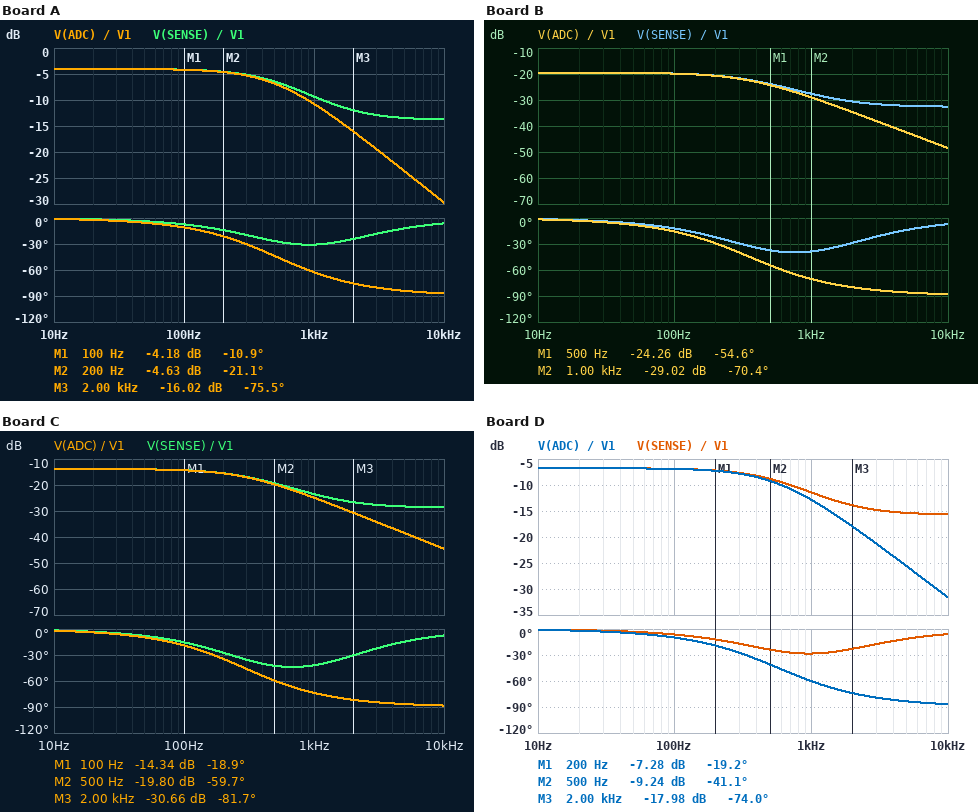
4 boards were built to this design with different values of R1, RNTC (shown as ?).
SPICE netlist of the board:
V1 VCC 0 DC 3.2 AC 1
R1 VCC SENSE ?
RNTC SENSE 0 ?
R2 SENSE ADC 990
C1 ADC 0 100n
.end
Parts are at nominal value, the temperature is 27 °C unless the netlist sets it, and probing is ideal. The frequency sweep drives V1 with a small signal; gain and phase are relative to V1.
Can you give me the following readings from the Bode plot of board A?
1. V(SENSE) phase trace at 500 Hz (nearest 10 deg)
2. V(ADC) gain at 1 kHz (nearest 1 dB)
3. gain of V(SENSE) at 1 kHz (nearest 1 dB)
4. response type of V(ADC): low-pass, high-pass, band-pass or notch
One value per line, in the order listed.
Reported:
-30 deg
-11 dB
-9 dB
low-pass
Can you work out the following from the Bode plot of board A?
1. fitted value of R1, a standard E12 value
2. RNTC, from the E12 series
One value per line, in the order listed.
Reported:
3.3 kΩ
5.6 kΩ
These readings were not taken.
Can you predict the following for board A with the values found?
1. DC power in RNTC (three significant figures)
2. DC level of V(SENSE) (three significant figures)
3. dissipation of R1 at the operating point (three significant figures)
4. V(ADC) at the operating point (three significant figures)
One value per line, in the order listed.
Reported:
724 µW
2.01 V
427 µW
2.01 V
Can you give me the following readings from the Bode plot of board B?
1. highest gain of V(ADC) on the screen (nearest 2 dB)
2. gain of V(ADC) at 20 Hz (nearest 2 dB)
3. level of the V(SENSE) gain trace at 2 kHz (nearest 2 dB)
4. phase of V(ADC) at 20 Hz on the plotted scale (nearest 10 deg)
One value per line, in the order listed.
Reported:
-20 dB
-20 dB
-30 dB
0 deg
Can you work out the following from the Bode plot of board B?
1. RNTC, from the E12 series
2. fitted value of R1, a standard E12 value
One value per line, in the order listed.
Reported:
3.9 kΩ
33 kΩ
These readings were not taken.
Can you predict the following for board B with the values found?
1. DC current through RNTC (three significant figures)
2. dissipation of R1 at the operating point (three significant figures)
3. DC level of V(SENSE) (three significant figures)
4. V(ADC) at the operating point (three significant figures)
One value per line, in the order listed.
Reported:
86.7 µA
248 µW
338 mV
338 mV
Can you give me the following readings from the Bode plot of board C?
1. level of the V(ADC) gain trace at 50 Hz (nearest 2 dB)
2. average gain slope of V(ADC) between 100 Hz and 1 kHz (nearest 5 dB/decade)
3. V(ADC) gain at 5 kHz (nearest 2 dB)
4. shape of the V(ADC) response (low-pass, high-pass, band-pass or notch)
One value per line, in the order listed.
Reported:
-14 dB
-10 dB/decade
-38 dB
low-pass
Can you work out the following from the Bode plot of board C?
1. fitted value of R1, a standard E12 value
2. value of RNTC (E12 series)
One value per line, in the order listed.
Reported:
22 kΩ
5.6 kΩ
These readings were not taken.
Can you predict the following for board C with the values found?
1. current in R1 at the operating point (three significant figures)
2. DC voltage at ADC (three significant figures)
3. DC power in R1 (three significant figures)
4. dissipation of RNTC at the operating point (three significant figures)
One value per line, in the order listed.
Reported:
116 µA
649 mV
296 µW
75.3 µW
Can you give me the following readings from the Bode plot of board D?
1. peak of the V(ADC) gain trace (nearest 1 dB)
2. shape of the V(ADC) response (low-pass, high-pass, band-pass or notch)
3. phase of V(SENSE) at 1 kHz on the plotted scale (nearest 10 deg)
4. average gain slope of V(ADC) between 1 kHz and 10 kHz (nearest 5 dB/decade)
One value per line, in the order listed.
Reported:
-7 dB
low-pass
-30 deg
-20 dB/decade
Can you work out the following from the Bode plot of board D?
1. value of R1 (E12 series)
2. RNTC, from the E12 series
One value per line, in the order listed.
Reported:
3.9 kΩ
3.3 kΩ
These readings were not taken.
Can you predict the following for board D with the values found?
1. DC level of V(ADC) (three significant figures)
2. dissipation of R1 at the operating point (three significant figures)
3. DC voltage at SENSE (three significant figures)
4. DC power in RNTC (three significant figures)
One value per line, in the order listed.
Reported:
1.47 V
770 µW
1.47 V
652 µW
